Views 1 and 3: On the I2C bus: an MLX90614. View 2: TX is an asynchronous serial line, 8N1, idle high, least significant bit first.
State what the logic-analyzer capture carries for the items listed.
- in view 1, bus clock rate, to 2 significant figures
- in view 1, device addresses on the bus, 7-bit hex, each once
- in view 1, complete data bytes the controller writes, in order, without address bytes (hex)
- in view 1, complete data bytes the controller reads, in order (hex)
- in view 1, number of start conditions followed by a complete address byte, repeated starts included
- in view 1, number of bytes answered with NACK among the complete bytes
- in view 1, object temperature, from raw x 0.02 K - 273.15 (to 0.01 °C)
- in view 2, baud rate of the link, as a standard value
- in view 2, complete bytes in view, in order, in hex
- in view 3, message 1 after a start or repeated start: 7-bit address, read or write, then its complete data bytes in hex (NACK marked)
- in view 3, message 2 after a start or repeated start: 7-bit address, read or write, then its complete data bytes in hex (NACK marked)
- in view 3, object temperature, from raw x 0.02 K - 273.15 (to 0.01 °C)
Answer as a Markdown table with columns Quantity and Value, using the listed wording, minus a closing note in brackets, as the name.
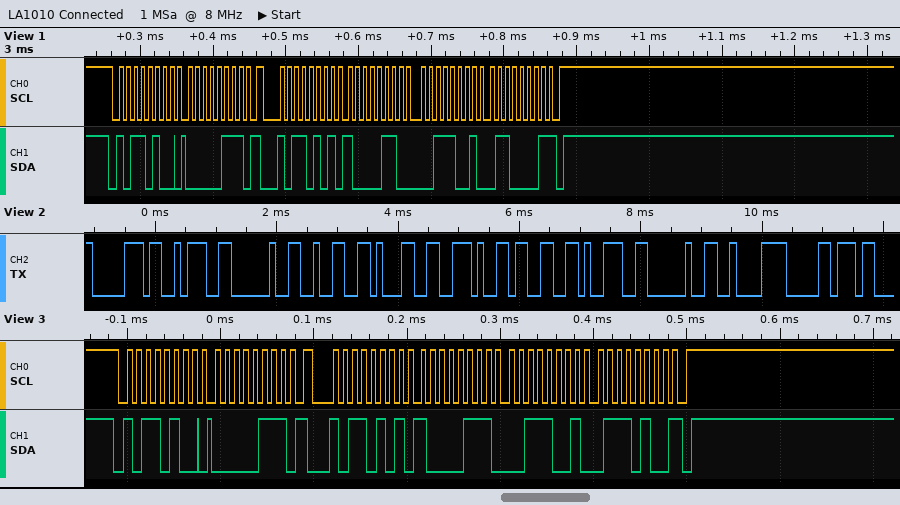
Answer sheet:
| Quantity | Value |
|---|---|
| in view 1, bus clock rate, to 2 significant figures | 100 kHz |
| in view 1, device addresses on the bus, 7-bit hex, each once | 0x5A |
| in view 1, complete data bytes the controller writes, in order, without address bytes | 07 |
| in view 1, complete data bytes the controller reads, in order | 86 39 61 |
| in view 1, number of start conditions followed by a complete address byte, repeated starts included | 2 |
| in view 1, number of bytes answered with NACK among the complete bytes | 1 |
| in view 1, object temperature, from raw x 0.02 K - 273.15 | 21.37 °C |
| in view 2, baud rate of the link, as a standard value | 9600 baud |
| in view 2, complete bytes in view, in order, in hex | 70 3A 20 32 31 2E 33 39 20 C2 B0 |
| in view 3, message 1 after a start or repeated start: 7-bit address, read or write, then its complete data bytes in hex | 0x5A write: 07 |
| in view 3, message 2 after a start or repeated start: 7-bit address, read or write, then its complete data bytes in hex | 0x5A read: 87 39 74 NACK |
| in view 3, object temperature, from raw x 0.02 K - 273.15 | 21.39 °C |
